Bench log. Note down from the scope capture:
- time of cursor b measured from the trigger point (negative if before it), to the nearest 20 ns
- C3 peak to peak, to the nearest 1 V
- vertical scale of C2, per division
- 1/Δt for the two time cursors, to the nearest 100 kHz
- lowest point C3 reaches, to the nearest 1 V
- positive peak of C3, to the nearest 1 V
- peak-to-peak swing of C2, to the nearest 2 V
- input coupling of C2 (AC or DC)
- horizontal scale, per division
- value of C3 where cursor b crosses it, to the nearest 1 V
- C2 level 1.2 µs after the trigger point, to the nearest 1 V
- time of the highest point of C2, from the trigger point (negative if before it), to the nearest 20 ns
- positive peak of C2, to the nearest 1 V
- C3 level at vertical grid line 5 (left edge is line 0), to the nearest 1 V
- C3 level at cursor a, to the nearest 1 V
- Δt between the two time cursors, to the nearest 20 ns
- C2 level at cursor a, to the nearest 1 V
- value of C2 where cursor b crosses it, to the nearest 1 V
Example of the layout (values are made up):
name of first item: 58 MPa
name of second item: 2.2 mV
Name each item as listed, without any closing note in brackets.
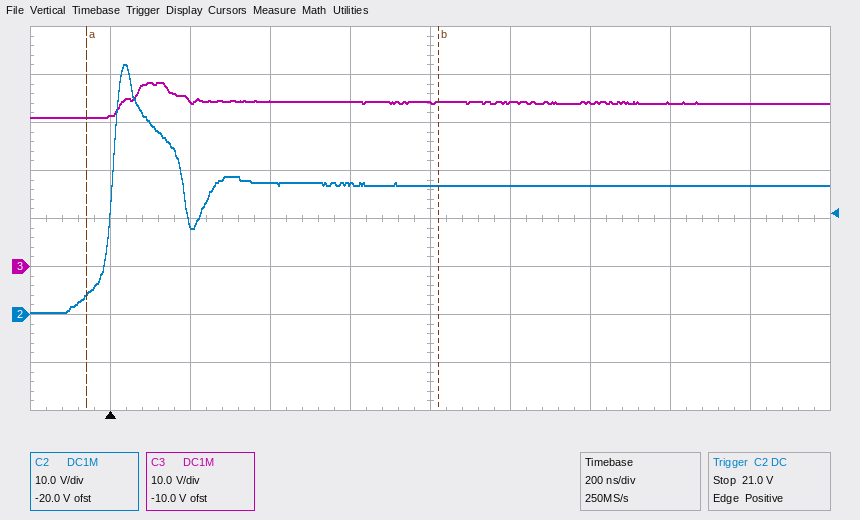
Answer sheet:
time of cursor b measured from the trigger point (negative if before it), to the nearest 20 ns: +820 ns
C3 peak to peak, to the nearest 1 V: 7 V
vertical scale of C2, per division: 10 V
1/Δt for the two time cursors, to the nearest 100 kHz: 1.1 MHz
lowest point C3 reaches, to the nearest 1 V: 31 V
positive peak of C3, to the nearest 1 V: 38 V
peak-to-peak swing of C2, to the nearest 2 V: 52 V
input coupling of C2: DC
horizontal scale, per division: 200 ns
value of C3 where cursor b crosses it, to the nearest 1 V: 34 V
C2 level 1.2 µs after the trigger point, to the nearest 1 V: 27 V
time of the highest point of C2, from the trigger point (negative if before it), to the nearest 20 ns: +40 ns
positive peak of C2, to the nearest 1 V: 52 V
C3 level at vertical grid line 5 (left edge is line 0), to the nearest 1 V: 34 V
C3 level at cursor a, to the nearest 1 V: 31 V
Δt between the two time cursors, to the nearest 20 ns: 880 ns
C2 level at cursor a, to the nearest 1 V: 4 V
value of C2 where cursor b crosses it, to the nearest 1 V: 27 V
